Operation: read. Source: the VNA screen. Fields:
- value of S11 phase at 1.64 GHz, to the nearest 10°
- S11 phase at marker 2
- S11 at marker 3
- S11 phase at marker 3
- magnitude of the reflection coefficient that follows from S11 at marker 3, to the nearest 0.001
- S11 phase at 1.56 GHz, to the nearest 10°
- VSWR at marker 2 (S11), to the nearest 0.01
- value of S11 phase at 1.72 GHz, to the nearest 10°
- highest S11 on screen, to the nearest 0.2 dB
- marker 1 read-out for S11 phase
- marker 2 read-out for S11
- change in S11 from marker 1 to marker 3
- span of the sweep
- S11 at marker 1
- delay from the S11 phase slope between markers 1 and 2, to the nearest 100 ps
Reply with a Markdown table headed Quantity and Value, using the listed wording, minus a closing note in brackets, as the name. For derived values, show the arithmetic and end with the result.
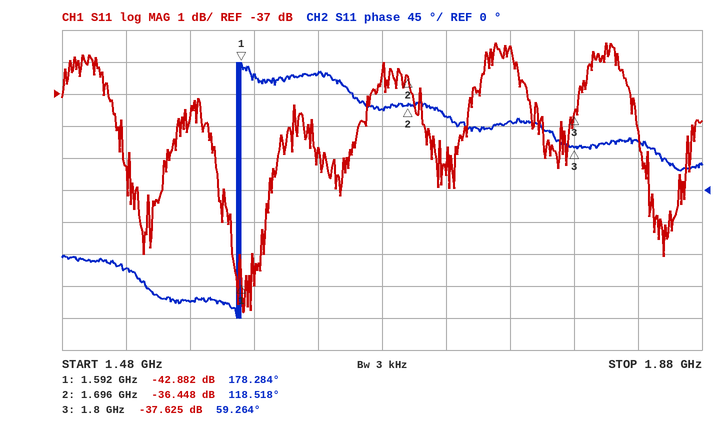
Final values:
| Quantity | Value |
|---|---|
| value of S11 phase at 1.64 GHz, to the nearest 10° | 160° |
| S11 phase at marker 2 | 118.518° |
| S11 at marker 3 | -37.625 dB |
| S11 phase at marker 3 | 59.264° |
| magnitude of the reflection coefficient that follows from S11 at marker 3, to the nearest 0.001 | 10^(-37.625/20) ≈ 0.013 |
| S11 phase at 1.56 GHz, to the nearest 10° | -160° |
| VSWR at marker 2 (S11), to the nearest 0.01 | (1 + 0.0151)/(1 − 0.0151) ≈ 1.03 |
| value of S11 phase at 1.72 GHz, to the nearest 10° | 100° |
| highest S11 on screen, to the nearest 0.2 dB | -35.4 dB |
| marker 1 read-out for S11 phase | 178.284° |
| marker 2 read-out for S11 | -36.448 dB |
| change in S11 from marker 1 to marker 3 | -37.625 − (-42.882) = 5.257 dB |
| span of the sweep | 400 MHz |
| S11 at marker 1 | -42.882 dB |
| delay from the S11 phase slope between markers 1 and 2, to the nearest 100 ps | −(118.518° − (178.284°))/(360° × 104 MHz) ≈ 1.6 ns |
